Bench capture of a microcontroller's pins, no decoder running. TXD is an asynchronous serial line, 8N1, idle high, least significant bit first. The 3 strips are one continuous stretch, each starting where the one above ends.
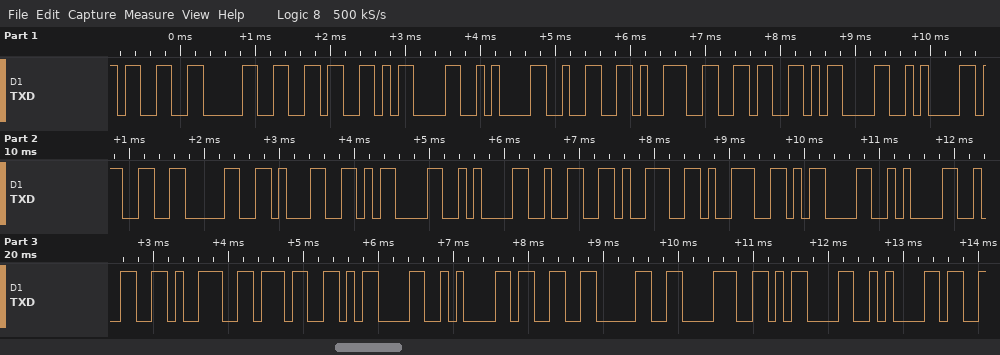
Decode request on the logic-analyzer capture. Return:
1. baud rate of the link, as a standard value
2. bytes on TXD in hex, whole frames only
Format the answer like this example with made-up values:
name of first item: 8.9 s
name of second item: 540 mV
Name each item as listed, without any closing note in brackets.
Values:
baud rate of the link, as a standard value: 9600 baud
bytes on TXD in hex, whole frames only: 33 30 36 0D 0A 32 39 36 0D 0A 33 30 31 0D 0A 32 39 39 0D 0A 32 39 37 0D 0A 33 30 38 0D 0A
